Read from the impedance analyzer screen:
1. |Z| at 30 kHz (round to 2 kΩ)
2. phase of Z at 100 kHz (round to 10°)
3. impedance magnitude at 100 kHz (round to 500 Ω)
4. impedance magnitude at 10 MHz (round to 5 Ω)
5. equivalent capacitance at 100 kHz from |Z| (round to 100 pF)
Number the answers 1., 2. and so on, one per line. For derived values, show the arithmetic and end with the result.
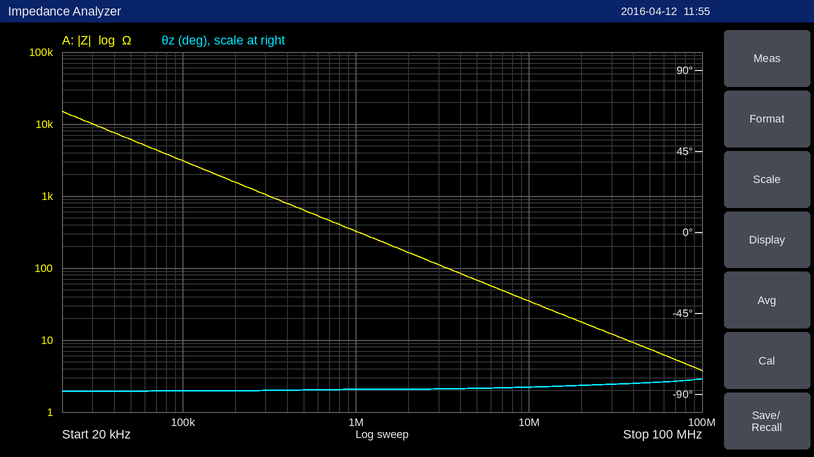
1. 10 kΩ
2. -90°
3. 3.0 kΩ
4. 35 Ω
5. C = 1/(2π × 100 kHz × 3.0 kΩ) ≈ 531 pF, so 500 pF to the nearest 100 pF
